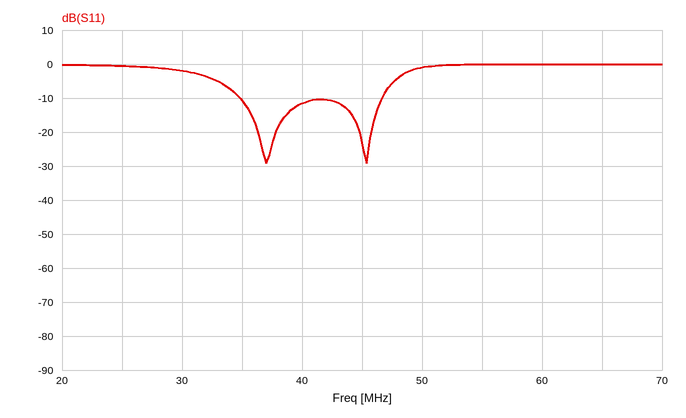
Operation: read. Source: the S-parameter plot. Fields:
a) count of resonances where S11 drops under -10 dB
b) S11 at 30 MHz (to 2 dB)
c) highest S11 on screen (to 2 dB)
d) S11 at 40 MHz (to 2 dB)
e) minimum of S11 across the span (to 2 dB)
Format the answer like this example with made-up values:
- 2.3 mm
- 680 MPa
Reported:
- 2
- -2 dB
- 0 dB
- -12 dB
- -30 dB
